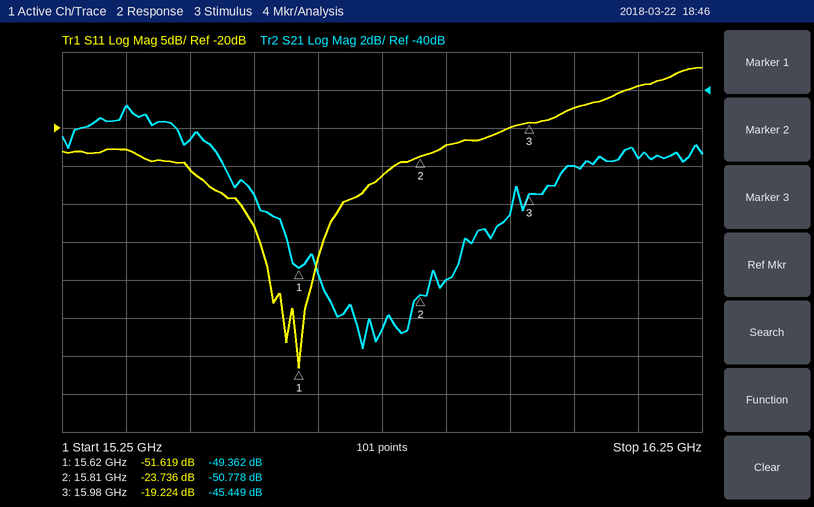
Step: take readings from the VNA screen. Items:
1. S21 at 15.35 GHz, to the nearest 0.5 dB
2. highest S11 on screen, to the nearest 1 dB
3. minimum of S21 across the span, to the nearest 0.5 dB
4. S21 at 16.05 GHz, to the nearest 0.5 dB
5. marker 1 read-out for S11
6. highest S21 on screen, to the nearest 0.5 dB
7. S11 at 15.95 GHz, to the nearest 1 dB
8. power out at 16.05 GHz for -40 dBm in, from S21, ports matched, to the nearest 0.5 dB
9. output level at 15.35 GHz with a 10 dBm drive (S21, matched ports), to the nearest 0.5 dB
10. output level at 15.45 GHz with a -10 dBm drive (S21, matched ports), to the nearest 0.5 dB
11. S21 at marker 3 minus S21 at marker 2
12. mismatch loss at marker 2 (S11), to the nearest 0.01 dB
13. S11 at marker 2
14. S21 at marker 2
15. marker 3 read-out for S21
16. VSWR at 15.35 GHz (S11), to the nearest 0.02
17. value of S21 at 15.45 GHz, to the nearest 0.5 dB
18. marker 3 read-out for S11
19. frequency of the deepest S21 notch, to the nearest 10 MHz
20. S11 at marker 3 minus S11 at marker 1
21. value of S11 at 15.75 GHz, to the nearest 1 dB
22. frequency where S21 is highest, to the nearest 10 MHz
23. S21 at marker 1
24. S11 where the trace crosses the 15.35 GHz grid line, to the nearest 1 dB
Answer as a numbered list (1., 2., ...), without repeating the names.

1. -41.0 dB
2. -12 dB
3. -53.5 dB
4. -44.0 dB
5. -51.619 dB
6. -41.0 dB
7. -20 dB
8. -84.0 dBm
9. -31.0 dBm
10. -52.5 dBm
11. 5.329 dB
12. 0.02 dB
13. -23.736 dB
14. -50.778 dB
15. -45.449 dB
16. 1.16
17. -42.5 dB
18. -19.224 dB
19. 15.72 GHz
20. 32.395 dB
21. -26 dB
22. 15.35 GHz
23. -49.362 dB
24. -23 dB
